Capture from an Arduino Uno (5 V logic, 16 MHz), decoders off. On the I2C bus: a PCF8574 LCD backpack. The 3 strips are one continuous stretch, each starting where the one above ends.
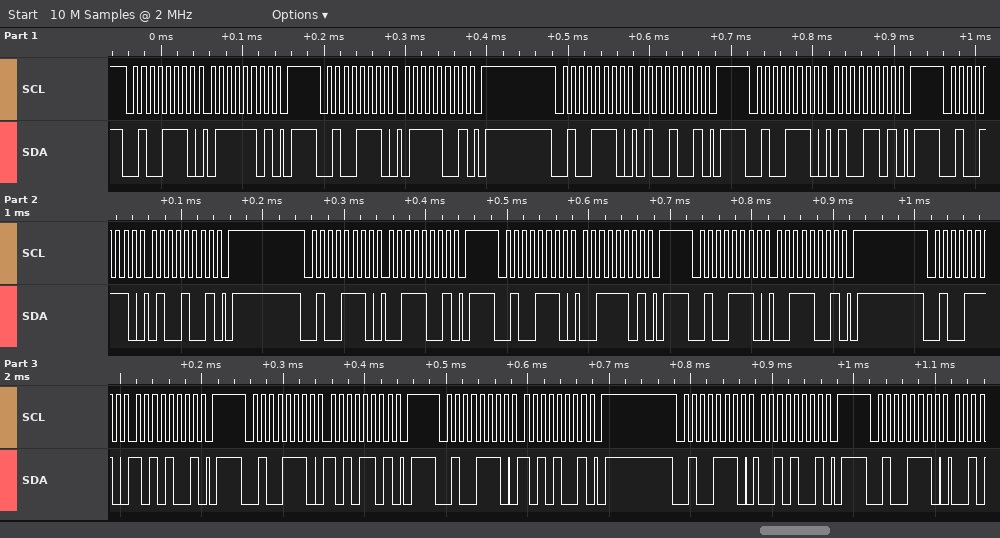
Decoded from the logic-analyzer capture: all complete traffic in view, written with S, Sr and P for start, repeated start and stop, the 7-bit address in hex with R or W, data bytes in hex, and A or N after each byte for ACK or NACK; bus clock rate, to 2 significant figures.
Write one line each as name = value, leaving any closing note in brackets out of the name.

all complete traffic in view, written with S, Sr and P for start, repeated start and stop, the 7-bit address in hex with R or W, data bytes in hex, and A or N after each byte for ACK or NACK = S 27W A 7D A P S 27W A 79 A P S 27W A 49 A P S 27W A 4D A P S 27W A 49 A P S 27W A 39 A P S 27W A 3D A P S 27W A 39 A P S 27W A A9 A P S 27W A AD A P S 27W A A9 A P S 27W A 29 A P S 27W A
bus clock rate, to 2 significant figures = 100 kHz
